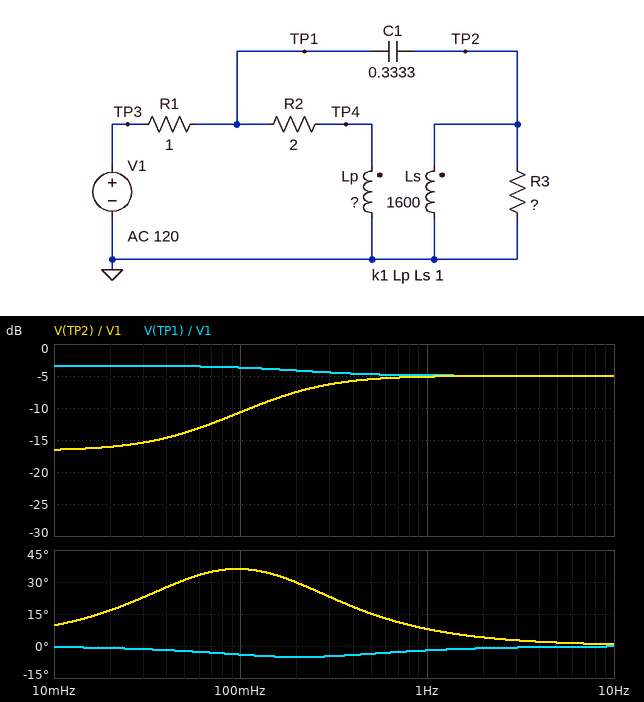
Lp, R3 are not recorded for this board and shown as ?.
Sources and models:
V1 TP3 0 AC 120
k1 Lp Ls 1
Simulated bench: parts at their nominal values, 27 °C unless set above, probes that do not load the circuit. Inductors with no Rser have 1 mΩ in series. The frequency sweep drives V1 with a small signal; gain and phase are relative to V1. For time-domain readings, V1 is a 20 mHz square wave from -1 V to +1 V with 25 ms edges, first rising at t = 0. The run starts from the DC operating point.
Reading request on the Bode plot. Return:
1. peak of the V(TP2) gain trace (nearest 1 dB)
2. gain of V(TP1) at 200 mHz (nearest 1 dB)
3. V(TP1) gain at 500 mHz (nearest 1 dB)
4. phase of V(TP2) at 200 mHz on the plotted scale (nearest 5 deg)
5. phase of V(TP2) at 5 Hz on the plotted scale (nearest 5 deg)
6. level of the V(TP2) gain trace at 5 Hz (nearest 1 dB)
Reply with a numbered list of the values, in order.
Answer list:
1. -5 dB
2. -4 dB
3. -5 dB
4. 30 deg
5. 0 deg
6. -5 dB
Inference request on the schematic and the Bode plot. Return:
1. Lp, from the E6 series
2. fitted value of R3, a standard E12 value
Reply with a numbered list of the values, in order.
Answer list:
1. 68 H
2. 2.2 Ω
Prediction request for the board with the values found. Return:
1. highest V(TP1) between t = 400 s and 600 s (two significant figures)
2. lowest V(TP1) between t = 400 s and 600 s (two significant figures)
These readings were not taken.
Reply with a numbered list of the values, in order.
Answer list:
1. 680 mV
2. -670 mV
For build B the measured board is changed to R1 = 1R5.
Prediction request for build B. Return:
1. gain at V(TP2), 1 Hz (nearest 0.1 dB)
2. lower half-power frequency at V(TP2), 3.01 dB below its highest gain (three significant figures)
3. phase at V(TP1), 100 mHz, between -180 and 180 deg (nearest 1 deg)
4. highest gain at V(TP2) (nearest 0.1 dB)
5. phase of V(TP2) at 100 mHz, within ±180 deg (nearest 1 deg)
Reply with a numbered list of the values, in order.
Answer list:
1. -6.8 dB
2. 167 mHz
3. -5 deg
4. -6.7 dB
5. 35 deg
